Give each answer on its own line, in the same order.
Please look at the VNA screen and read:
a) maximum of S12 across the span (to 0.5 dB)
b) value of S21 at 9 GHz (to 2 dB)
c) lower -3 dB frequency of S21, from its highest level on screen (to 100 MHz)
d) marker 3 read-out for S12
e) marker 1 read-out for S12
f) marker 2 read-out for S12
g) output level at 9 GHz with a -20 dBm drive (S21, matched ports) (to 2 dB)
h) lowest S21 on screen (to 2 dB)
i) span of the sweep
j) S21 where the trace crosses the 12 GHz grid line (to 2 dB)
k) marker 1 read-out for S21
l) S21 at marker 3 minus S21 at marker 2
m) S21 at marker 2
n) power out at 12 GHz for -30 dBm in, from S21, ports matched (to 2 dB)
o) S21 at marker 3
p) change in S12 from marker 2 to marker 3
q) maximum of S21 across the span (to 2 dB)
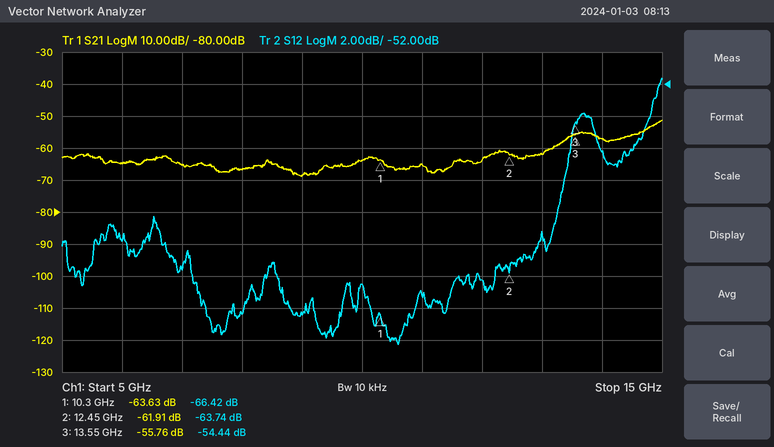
-51.5 dB
-68 dB
14.7 GHz
-54.44 dB
-66.42 dB
-63.74 dB
-88 dBm
-68 dB
10 GHz
-64 dB
-63.63 dB
6.15 dB
-61.91 dB
-94 dBm
-55.76 dB
9.30 dB
-52 dB
